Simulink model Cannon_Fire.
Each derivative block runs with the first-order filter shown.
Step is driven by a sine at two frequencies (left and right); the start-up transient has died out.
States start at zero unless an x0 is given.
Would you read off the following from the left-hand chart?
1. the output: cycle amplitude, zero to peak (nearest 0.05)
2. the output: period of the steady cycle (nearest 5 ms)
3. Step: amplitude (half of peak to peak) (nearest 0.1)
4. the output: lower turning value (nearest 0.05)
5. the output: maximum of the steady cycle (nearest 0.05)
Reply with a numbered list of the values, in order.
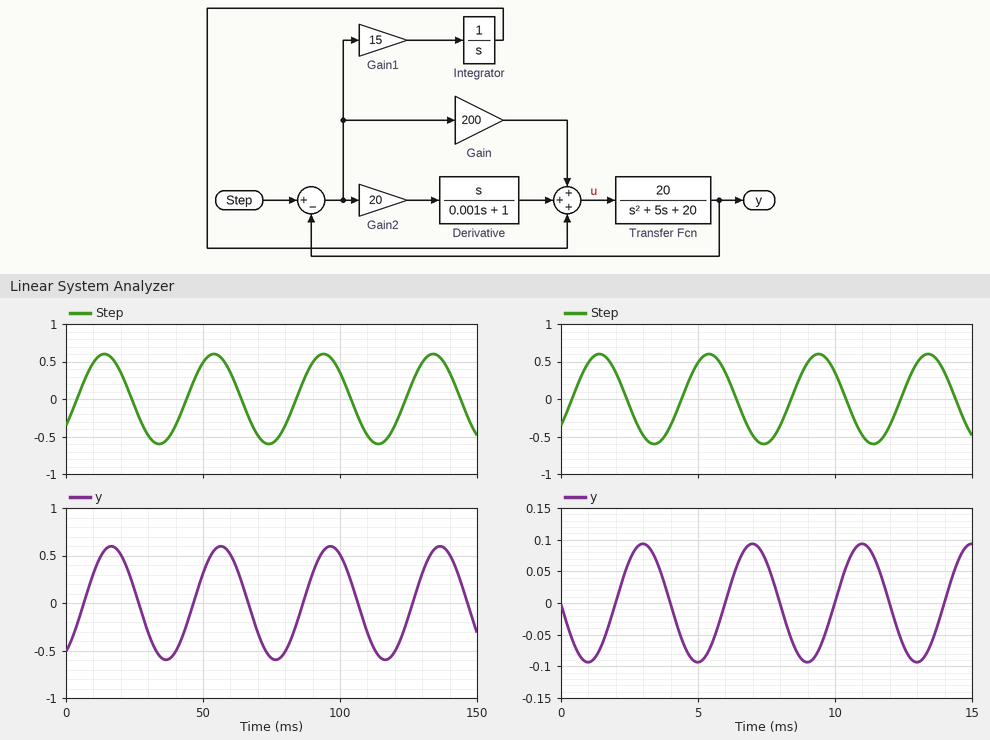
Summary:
1. 0.60
2. 40 ms
3. 0.6
4. -0.60
5. 0.60
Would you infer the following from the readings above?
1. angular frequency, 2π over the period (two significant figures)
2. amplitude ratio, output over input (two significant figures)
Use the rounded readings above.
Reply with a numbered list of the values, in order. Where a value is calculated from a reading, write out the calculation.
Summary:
1. 2π / 40 = 0.16 rad/ms
2. 0.6 / 0.6 = 1.0
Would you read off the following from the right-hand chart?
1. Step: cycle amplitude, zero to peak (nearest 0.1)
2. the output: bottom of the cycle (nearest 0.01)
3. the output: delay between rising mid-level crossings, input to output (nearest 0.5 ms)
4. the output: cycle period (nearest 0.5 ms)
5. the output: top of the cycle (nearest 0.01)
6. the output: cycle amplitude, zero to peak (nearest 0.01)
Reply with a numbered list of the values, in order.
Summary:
1. 0.6
2. -0.09
3. 1.5 ms
4. 4.0 ms
5. 0.09
6. 0.09
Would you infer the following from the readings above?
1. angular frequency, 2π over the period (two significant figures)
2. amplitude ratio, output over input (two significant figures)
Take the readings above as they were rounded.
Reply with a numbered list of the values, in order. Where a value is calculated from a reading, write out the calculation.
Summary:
1. 2π / 4 = 1.6 rad/ms
2. 0.09 / 0.6 = 0.15
